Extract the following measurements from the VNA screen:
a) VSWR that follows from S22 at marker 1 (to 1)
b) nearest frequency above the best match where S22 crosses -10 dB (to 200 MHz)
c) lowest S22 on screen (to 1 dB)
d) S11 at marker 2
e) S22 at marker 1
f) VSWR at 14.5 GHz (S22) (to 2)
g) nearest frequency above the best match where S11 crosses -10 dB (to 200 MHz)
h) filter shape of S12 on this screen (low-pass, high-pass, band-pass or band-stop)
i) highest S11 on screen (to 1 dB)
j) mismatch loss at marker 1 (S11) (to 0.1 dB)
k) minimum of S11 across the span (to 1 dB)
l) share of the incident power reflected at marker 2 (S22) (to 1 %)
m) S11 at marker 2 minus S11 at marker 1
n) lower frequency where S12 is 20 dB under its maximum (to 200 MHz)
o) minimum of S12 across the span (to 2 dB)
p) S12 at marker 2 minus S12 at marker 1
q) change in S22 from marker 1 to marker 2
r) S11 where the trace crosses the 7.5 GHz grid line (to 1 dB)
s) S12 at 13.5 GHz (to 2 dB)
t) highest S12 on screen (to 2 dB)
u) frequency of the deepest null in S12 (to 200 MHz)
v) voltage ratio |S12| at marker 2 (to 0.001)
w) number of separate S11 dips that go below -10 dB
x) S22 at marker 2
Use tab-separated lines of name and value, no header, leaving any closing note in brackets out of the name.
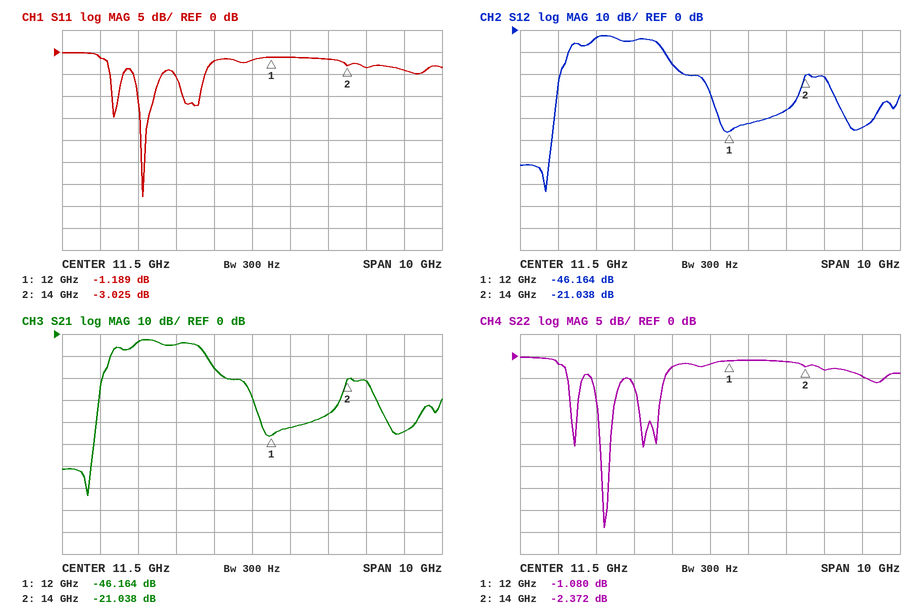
VSWR that follows from S22 at marker 1	16
nearest frequency above the best match where S22 crosses -10 dB	9.0 GHz
lowest S22 on screen	-39 dB
S11 at marker 2	-3.025 dB
S22 at marker 1	-1.080 dB
VSWR at 14.5 GHz (S22)	6
nearest frequency above the best match where S11 crosses -10 dB	9.0 GHz
filter shape of S12 on this screen	band-pass
highest S11 on screen	0 dB
mismatch loss at marker 1 (S11)	6.2 dB
minimum of S11 across the span	-33 dB
share of the incident power reflected at marker 2 (S22)	58 %
S11 at marker 2 minus S11 at marker 1	-1.836 dB
lower frequency where S12 is 20 dB under its maximum	7.6 GHz
minimum of S12 across the span	-74 dB
S12 at marker 2 minus S12 at marker 1	25.126 dB
change in S22 from marker 1 to marker 2	-1.292 dB
S11 where the trace crosses the 7.5 GHz grid line	-1 dB
S12 at 13.5 GHz	-36 dB
highest S12 on screen	-2 dB
frequency of the deepest null in S12	7.2 GHz
voltage ratio |S12| at marker 2	0.089
number of separate S11 dips that go below -10 dB	3
S22 at marker 2	-2.372 dB
